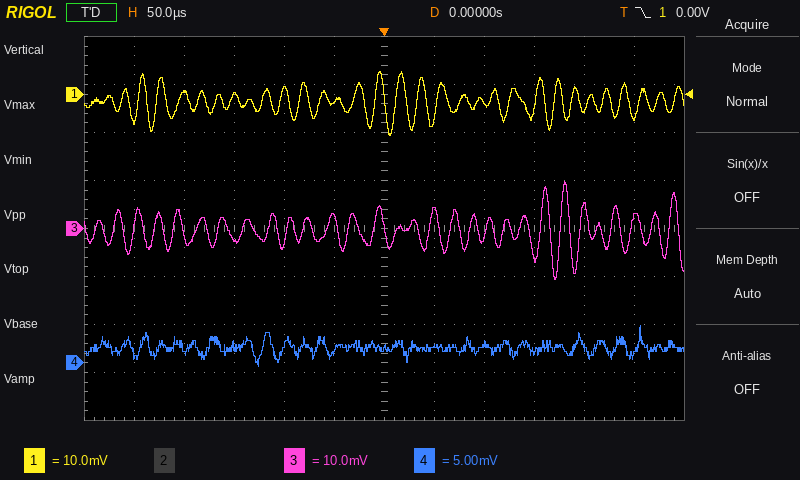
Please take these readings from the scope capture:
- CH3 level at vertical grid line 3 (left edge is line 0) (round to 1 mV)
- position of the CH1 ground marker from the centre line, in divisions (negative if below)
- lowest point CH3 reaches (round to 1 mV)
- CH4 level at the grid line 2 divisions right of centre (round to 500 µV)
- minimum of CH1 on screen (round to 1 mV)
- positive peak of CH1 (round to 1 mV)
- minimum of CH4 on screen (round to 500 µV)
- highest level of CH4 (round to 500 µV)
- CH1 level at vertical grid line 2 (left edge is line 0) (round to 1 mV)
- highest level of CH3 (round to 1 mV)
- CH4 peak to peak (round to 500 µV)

-2 mV
+2.8 div
-11 mV
2.0 mV
-9 mV
5 mV
-500 µV
4.0 mV
0 mV
10 mV
4.5 mV
